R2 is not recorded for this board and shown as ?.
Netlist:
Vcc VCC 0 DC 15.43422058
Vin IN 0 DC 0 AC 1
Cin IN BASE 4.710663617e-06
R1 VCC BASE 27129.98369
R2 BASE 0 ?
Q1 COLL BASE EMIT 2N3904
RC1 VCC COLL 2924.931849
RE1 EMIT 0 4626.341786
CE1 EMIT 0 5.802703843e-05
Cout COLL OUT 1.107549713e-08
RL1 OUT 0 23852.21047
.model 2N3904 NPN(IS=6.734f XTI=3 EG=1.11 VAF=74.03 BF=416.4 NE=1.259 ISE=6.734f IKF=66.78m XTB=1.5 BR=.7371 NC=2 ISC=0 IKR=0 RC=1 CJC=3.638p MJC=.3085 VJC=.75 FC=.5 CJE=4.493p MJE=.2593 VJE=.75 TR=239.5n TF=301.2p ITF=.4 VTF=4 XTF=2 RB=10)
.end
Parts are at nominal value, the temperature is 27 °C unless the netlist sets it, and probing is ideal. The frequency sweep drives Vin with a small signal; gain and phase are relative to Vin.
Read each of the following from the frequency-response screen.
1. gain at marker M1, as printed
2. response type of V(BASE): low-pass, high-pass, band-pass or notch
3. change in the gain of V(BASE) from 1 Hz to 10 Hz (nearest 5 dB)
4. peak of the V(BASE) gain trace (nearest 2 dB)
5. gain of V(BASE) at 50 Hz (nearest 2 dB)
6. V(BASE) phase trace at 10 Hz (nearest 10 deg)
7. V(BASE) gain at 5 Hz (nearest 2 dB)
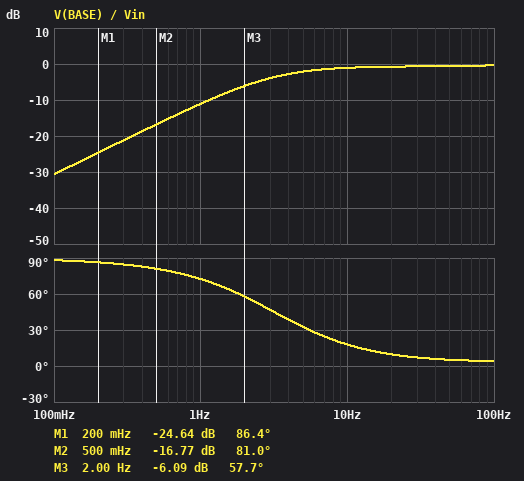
-24.64 dB
high-pass
10 dB
0 dB
0 dB
20 deg
-2 dB
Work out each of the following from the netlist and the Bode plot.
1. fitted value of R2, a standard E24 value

16 kΩ
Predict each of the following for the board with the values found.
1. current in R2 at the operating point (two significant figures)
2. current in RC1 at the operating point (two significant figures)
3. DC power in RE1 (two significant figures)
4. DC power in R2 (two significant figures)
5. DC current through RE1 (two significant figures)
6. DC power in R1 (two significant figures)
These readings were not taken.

350 µA
1.1 mA
5.4 mW
2.0 mW
1.1 mA
3.5 mW
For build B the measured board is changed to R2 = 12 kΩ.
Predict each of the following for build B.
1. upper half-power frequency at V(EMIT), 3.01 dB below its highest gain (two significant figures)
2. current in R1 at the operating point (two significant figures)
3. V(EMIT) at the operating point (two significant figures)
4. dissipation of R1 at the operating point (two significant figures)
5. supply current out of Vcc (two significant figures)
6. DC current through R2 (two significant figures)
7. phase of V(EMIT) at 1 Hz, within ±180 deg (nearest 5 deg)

100 Hz
400 µA
4.0 V
4.3 mW
1.3 mA
390 µA
75 deg
